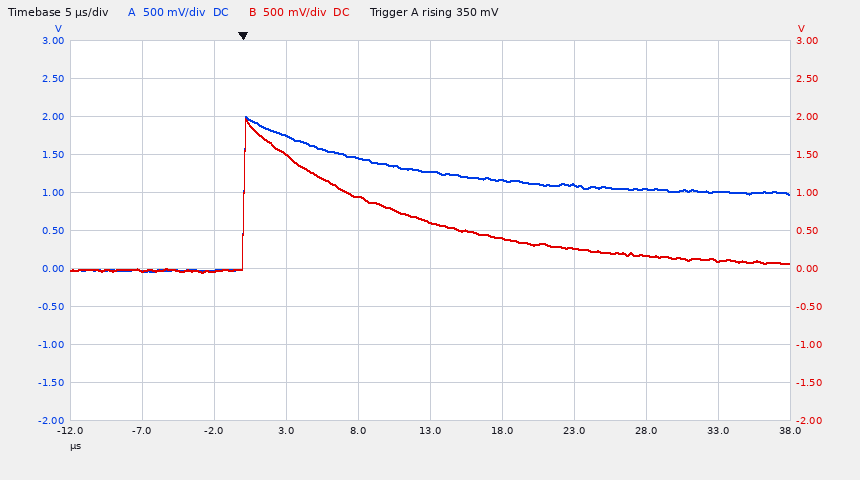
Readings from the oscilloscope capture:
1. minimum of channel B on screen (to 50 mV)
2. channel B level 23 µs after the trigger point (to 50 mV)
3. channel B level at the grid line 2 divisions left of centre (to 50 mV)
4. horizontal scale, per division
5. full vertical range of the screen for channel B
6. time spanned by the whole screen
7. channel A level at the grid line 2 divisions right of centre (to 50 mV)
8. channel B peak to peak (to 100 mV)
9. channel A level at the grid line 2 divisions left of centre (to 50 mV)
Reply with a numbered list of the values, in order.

1. -50 mV
2. 250 mV
3. 1.50 V
4. 5 µs
5. 5 V
6. 50 µs
7. 1.10 V
8. 2.00 V
9. 1.75 V
